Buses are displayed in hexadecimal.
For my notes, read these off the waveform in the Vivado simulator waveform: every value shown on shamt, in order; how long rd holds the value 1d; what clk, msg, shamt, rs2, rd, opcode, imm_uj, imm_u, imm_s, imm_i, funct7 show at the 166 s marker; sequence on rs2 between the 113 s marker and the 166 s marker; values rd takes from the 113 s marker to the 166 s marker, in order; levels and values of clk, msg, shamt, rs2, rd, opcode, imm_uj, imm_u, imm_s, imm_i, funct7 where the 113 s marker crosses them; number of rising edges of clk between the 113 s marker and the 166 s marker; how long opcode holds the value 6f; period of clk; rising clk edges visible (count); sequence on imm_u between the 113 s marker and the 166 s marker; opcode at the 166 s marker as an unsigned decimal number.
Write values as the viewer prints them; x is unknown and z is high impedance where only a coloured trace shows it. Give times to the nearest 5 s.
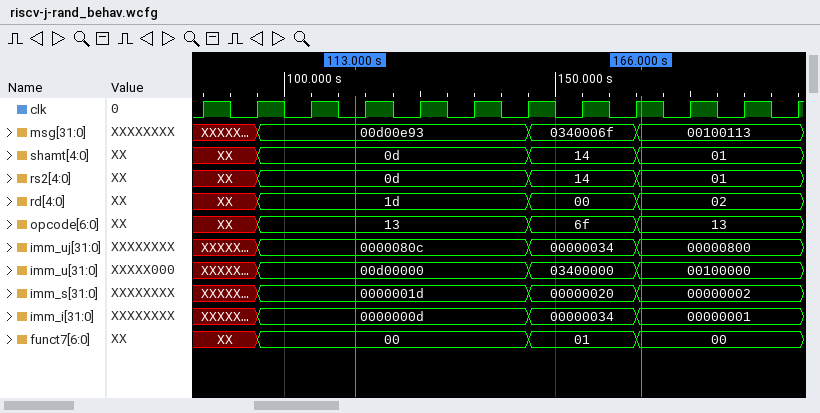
XX, 0d, 14, 01
50 s
clk=1, msg=00100113, shamt=01, rs2=01, rd=02, opcode=13, imm_uj=00000800, imm_u=00100000, imm_s=00000002, imm_i=00000001, funct7=00
0d, 14, 01
1d, 00, 02
clk=0, msg=00d00e93, shamt=0d, rs2=0d, rd=1d, opcode=13, imm_uj=0000080c, imm_u=00d00000, imm_s=0000001d, imm_i=0000000d, funct7=00
6
20 s
10 s
12
00d00000, 03400000, 00100000
19
